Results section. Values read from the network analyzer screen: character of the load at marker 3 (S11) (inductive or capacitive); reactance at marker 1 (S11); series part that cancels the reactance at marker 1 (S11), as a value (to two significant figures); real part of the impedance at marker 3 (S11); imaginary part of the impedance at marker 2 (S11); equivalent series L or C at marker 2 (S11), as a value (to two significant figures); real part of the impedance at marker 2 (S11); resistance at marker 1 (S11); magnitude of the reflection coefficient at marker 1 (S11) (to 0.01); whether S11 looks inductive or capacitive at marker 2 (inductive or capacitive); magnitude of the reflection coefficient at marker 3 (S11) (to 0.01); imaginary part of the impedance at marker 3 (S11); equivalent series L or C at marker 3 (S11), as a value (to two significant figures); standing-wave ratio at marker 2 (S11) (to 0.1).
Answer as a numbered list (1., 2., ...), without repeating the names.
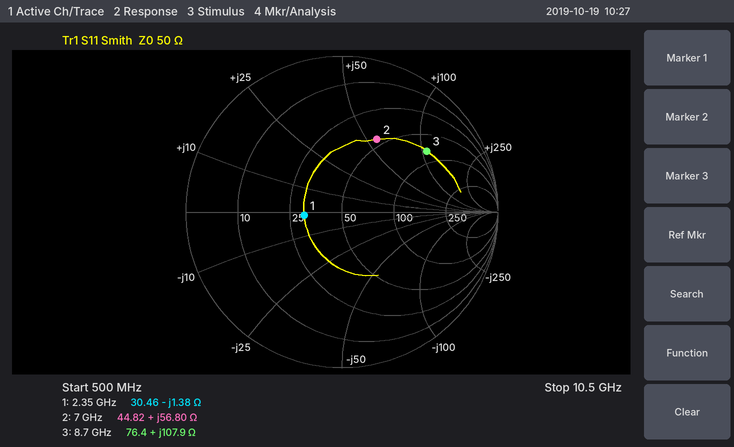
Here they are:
1. inductive
2. -1.38 Ω
3. 93 pH
4. 76.4 Ω
5. +56.80 Ω
6. 1.3 nH
7. 44.82 Ω
8. 30.46 Ω
9. 0.24
10. inductive
11. 0.67
12. +107.9 Ω
13. 2.0 nH
14. 3.1
